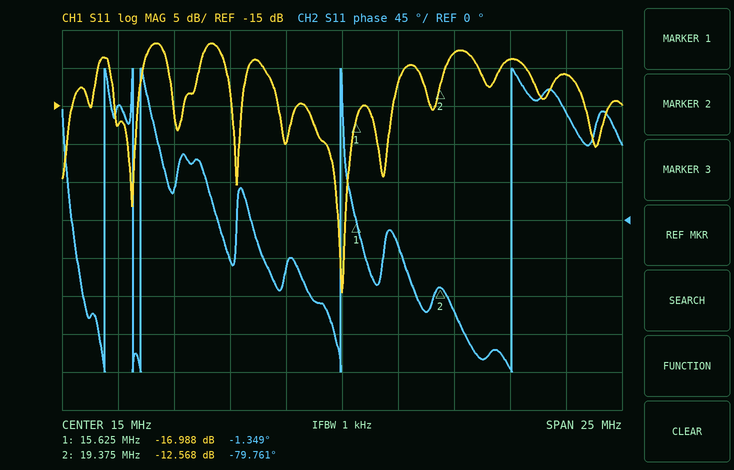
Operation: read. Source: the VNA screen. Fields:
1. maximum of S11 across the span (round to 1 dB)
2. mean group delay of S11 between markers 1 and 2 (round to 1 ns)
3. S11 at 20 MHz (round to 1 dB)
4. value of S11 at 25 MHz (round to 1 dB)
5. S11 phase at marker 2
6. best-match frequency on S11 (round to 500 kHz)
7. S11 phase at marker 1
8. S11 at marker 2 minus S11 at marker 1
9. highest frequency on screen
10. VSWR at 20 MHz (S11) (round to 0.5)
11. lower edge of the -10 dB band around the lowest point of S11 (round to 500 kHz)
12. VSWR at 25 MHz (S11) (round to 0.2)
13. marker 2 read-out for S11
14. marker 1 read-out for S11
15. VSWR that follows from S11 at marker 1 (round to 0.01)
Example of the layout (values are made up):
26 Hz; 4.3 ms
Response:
-7 dB; 58 ns; -8 dB; -11 dB; -79.761°; 15.0 MHz; -1.349°; 4.420 dB; 27.5 MHz; 2.5; 11.5 MHz; 1.8; -12.568 dB; -16.988 dB; 1.33
